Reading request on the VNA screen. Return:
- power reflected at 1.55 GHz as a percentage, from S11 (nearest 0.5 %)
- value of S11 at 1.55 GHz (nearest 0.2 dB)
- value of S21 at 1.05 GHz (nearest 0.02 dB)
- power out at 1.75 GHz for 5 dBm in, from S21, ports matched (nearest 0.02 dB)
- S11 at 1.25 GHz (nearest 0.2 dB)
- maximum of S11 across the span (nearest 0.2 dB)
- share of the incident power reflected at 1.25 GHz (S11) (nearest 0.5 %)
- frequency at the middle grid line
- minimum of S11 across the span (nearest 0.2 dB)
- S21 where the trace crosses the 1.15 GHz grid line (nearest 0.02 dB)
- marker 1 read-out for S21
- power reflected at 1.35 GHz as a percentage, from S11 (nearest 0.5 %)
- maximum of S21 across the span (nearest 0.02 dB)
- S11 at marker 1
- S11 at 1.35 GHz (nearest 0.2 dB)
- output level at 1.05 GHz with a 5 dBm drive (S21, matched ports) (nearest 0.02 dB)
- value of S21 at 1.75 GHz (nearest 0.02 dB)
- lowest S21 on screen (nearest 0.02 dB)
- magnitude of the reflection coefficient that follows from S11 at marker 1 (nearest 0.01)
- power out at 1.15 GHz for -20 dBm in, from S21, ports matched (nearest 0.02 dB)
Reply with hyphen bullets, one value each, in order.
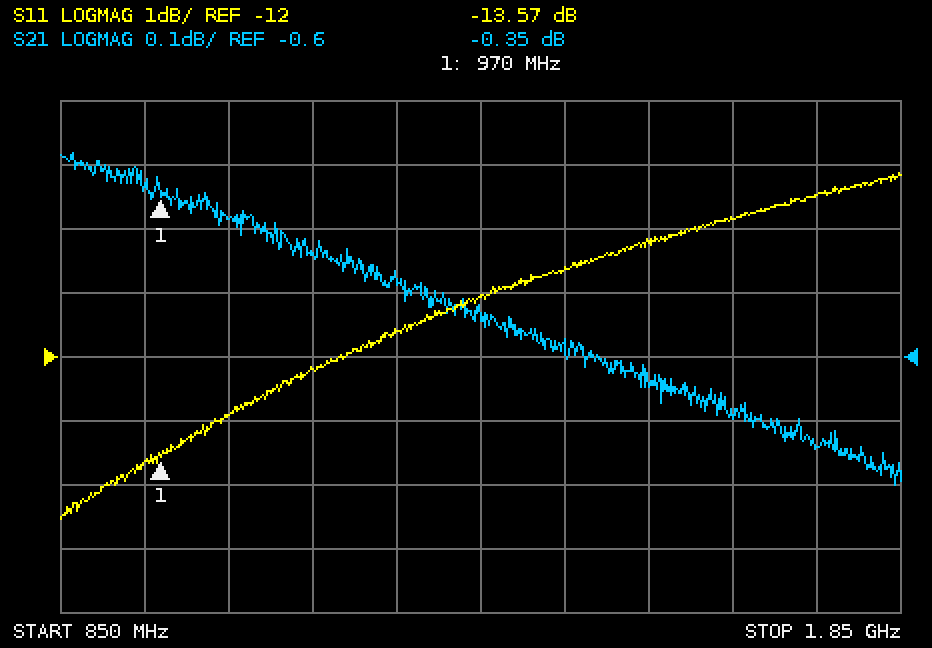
- 9.5 %
- -10.2 dB
- -0.38 dB
- 4.26 dBm
- -11.6 dB
- -9.2 dB
- 7.0 %
- 1.35 GHz
- -14.6 dB
- -0.44 dB
- -0.35 dB
- 8.0 %
- -0.28 dB
- -13.57 dB
- -11.0 dB
- 4.62 dBm
- -0.74 dB
- -0.80 dB
- 0.21
- -20.44 dBm
